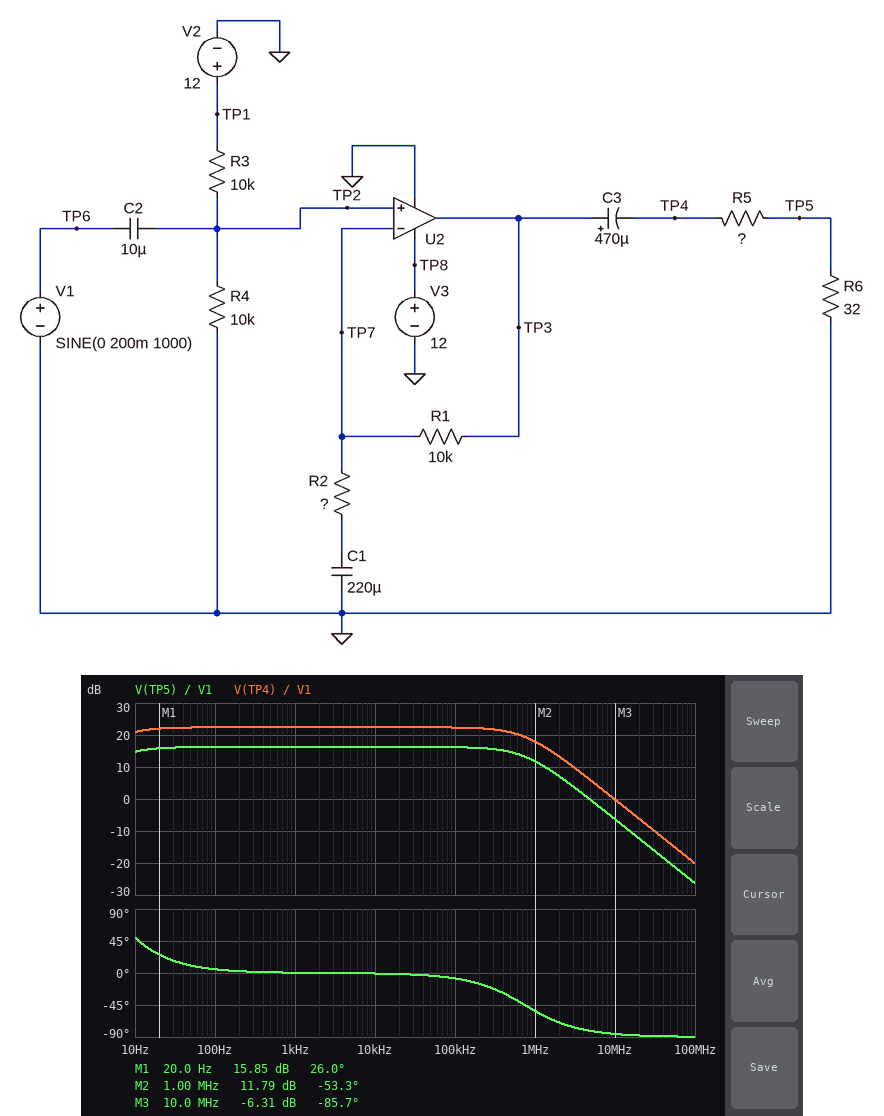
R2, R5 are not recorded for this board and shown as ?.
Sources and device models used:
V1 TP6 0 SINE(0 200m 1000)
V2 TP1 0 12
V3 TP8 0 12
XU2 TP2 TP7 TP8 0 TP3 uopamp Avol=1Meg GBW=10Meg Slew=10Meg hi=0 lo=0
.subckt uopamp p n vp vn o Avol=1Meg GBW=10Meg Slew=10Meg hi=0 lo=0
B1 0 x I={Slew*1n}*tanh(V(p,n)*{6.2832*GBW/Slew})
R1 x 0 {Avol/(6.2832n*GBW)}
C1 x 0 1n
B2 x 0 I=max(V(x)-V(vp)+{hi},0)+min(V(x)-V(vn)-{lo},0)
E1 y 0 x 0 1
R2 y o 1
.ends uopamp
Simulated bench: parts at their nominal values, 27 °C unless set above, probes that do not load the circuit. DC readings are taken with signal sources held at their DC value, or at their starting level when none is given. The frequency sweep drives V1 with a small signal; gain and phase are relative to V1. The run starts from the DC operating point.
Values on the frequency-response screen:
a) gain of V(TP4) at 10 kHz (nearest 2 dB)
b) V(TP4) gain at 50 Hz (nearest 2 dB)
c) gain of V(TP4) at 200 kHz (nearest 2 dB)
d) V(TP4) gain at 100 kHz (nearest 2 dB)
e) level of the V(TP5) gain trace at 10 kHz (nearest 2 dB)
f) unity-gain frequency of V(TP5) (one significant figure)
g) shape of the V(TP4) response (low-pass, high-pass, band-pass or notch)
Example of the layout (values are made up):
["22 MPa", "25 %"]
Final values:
["22 dB", "22 dB", "22 dB", "22 dB", "16 dB", "5 MHz", "low-pass"]
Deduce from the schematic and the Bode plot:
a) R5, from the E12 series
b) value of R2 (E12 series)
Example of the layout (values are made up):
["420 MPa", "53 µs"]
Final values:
["33 Ω", "820 Ω"]
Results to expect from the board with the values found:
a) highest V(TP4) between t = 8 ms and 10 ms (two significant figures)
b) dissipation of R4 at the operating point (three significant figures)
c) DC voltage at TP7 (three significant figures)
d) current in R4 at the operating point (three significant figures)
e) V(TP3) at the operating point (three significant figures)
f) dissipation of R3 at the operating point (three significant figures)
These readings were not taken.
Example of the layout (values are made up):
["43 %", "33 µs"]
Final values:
["2.6 V", "3.60 mW", "6.00 V", "600 µA", "6.00 V", "3.60 mW"]
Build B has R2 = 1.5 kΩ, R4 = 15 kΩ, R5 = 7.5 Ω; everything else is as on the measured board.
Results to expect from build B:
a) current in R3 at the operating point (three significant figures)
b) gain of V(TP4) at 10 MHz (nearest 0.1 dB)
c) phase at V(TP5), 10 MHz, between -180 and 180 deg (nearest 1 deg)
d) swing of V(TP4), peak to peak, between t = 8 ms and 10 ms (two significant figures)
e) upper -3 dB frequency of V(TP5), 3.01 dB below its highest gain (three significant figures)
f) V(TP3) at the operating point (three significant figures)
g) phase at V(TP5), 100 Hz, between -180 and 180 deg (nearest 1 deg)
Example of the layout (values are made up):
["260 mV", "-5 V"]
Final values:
["480 µA", "-0.3 dB", "-83 deg", "3.1 V", "1.27 MHz", "7.20 V", "7 deg"]
